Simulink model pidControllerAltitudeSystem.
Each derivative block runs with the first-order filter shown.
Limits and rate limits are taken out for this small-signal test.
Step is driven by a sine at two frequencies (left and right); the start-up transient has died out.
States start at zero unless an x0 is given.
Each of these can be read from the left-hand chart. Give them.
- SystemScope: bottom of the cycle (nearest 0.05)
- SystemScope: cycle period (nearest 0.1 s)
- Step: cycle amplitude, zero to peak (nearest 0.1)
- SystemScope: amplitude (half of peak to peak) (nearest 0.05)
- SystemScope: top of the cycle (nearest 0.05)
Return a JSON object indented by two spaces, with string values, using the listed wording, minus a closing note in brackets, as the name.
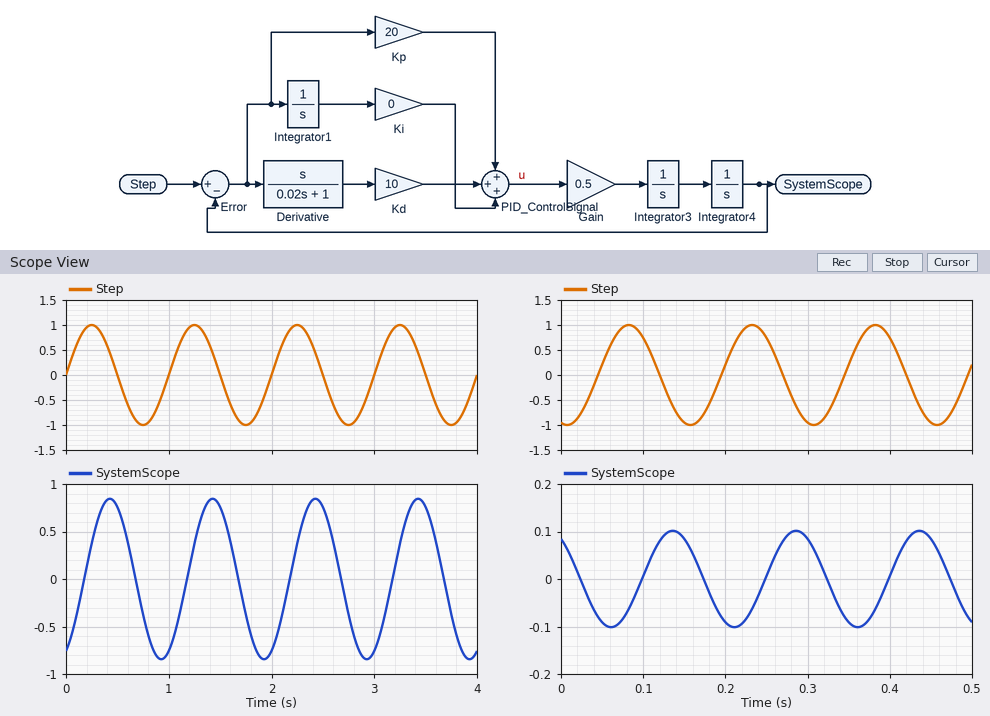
{
  "SystemScope: bottom of the cycle": "-0.85",
  "SystemScope: cycle period": "1.0 s",
  "Step: cycle amplitude, zero to peak": "1.0",
  "SystemScope: amplitude (half of peak to peak)": "0.85",
  "SystemScope: top of the cycle": "0.85"
}
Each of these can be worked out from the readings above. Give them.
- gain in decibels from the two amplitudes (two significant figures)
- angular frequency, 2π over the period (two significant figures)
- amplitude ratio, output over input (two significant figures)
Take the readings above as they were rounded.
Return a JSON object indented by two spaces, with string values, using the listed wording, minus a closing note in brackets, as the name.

{
  "gain in decibels from the two amplitudes": "-1.4 dB",
  "angular frequency, 2π over the period": "6.3 rad/s",
  "amplitude ratio, output over input": "0.85"
}
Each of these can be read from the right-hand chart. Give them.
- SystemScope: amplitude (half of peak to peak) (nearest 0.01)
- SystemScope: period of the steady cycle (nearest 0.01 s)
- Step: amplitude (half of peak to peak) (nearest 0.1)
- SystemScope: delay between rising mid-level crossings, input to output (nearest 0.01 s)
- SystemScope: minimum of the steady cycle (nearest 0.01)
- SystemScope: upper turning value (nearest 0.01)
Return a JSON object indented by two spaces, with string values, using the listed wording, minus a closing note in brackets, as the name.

{
  "SystemScope: amplitude (half of peak to peak)": "0.10",
  "SystemScope: period of the steady cycle": "0.15 s",
  "Step: amplitude (half of peak to peak)": "1.0",
  "SystemScope: delay between rising mid-level crossings, input to output": "0.05 s",
  "SystemScope: minimum of the steady cycle": "-0.10",
  "SystemScope: upper turning value": "0.10"
}
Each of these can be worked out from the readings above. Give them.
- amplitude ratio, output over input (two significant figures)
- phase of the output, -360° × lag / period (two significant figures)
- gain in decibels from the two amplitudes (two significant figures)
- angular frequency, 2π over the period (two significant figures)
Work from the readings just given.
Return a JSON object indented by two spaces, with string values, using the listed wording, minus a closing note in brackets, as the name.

{
  "amplitude ratio, output over input": "0.10",
  "phase of the output, -360° × lag / period": "-120°",
  "gain in decibels from the two amplitudes": "-20 dB",
  "angular frequency, 2π over the period": "42 rad/s"
}
